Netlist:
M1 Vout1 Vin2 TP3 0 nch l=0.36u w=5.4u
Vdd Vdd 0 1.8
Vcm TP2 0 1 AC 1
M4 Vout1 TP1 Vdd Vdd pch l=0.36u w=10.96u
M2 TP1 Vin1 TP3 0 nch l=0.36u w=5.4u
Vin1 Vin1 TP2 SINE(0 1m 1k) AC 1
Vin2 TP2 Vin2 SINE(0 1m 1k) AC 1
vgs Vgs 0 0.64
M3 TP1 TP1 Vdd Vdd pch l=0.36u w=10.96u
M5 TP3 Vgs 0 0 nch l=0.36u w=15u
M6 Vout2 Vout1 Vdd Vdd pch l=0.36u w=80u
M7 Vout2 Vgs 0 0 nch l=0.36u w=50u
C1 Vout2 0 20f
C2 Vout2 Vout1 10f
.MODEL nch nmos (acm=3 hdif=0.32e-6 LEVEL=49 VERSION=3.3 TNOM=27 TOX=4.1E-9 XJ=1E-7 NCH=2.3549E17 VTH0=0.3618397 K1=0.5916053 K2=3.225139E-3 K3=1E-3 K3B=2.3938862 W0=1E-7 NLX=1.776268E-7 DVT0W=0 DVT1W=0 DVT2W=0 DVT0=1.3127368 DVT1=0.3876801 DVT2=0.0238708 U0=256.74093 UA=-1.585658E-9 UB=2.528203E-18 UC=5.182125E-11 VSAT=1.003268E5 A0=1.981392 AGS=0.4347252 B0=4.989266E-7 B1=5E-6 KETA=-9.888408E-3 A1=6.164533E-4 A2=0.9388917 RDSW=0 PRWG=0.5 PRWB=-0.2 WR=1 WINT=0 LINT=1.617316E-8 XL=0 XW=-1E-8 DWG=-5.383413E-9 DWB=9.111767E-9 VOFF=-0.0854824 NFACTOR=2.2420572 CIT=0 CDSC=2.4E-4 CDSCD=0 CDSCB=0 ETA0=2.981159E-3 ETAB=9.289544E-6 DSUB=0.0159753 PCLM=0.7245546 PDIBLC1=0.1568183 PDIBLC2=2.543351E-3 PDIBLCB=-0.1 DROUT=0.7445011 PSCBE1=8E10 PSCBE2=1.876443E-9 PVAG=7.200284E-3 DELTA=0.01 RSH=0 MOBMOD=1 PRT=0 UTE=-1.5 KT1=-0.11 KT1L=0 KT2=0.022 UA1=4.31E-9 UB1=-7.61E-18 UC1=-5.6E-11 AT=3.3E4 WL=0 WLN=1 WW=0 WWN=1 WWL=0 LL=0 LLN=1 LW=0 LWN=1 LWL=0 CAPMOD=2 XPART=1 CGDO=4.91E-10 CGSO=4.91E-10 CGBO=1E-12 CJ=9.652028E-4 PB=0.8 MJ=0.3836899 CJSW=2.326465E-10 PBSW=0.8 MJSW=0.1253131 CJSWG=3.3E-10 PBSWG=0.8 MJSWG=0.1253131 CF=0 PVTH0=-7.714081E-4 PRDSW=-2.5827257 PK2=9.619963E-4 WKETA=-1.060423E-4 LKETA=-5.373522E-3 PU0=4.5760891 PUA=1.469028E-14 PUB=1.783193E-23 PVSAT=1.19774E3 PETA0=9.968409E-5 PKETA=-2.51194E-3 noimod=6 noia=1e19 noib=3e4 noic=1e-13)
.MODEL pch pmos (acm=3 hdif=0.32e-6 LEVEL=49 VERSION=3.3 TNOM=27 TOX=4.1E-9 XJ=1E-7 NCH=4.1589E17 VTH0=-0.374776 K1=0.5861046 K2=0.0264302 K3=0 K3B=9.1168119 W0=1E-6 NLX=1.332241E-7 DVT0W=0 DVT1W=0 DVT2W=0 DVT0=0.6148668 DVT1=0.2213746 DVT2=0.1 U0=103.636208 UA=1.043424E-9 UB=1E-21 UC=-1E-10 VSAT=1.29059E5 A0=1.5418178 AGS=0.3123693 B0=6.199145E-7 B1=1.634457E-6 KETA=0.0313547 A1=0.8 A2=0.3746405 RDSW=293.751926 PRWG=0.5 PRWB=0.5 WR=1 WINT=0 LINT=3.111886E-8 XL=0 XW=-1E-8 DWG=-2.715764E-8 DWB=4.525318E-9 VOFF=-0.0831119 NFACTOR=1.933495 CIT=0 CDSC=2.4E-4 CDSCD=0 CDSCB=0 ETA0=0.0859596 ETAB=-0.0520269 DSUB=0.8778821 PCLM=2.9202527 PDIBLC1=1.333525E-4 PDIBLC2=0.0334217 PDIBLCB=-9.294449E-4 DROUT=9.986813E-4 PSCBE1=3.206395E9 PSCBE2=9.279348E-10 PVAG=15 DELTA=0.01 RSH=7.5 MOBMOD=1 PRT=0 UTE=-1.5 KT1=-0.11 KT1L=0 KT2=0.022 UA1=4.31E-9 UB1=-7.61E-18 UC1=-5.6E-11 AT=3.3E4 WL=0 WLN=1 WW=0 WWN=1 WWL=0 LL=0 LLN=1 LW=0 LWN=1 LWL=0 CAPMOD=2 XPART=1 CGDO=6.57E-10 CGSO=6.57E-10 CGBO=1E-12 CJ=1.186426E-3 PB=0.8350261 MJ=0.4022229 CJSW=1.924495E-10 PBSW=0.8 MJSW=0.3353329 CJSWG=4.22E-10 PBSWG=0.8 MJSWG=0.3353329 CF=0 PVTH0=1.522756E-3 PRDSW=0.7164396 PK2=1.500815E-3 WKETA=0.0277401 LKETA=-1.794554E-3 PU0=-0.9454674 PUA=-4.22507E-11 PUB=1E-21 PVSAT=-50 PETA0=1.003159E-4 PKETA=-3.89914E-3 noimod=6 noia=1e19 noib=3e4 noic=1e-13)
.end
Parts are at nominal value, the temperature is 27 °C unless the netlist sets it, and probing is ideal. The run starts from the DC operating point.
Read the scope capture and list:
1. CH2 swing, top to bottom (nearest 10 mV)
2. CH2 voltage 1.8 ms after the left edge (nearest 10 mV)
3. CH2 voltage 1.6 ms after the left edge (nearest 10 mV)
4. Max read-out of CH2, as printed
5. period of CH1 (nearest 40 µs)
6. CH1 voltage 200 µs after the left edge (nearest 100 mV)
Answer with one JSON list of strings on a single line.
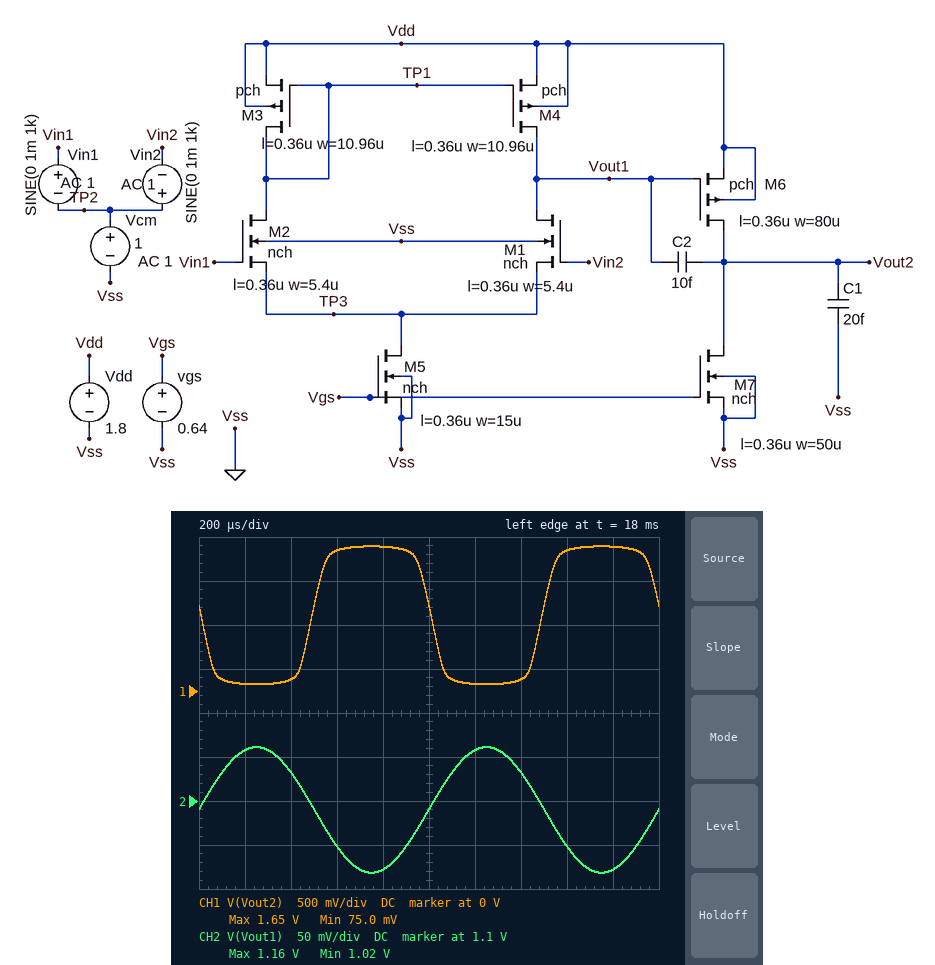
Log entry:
["140 mV", "1.02 V", "1.05 V", "1.16 V", "1.00 ms", "100 mV"]
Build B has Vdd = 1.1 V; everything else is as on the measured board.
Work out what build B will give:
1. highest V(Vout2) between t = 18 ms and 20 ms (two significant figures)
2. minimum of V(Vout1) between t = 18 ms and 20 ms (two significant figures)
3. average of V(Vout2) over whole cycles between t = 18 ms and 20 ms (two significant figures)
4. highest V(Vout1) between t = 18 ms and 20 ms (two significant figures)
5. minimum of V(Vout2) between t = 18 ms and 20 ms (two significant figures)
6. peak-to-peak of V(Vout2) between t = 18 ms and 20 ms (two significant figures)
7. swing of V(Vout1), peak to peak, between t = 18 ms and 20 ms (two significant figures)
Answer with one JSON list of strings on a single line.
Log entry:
["680 mV", "390 mV", "570 mV", "400 mV", "450 mV", "230 mV", "11 mV"]
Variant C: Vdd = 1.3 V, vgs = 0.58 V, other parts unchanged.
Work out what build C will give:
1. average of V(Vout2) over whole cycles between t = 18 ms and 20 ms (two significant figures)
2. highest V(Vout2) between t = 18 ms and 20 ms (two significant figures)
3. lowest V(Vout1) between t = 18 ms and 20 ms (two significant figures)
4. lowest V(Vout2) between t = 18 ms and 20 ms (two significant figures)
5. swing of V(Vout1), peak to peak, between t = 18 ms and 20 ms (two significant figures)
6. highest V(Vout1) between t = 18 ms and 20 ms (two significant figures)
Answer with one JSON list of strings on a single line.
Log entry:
["640 mV", "1.2 V", "610 mV", "38 mV", "130 mV", "750 mV"]
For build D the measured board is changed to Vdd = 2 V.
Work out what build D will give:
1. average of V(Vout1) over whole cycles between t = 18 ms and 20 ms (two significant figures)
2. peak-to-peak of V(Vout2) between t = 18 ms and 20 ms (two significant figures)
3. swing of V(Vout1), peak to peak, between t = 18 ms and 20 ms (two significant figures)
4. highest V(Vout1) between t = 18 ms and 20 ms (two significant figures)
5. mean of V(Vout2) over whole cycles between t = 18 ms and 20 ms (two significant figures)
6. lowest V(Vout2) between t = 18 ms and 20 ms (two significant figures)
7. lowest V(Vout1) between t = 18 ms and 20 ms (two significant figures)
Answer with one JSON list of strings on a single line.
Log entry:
["1.3 V", "1.8 V", "150 mV", "1.4 V", "980 mV", "78 mV", "1.2 V"]
